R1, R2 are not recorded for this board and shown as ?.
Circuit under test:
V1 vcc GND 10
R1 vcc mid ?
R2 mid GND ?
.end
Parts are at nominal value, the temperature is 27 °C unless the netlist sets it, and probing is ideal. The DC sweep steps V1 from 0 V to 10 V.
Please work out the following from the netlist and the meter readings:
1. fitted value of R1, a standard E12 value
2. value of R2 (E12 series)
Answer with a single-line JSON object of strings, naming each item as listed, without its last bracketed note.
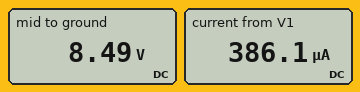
{"fitted value of R1, a standard E12 value": "3.9 kΩ", "value of R2": "22 kΩ"}
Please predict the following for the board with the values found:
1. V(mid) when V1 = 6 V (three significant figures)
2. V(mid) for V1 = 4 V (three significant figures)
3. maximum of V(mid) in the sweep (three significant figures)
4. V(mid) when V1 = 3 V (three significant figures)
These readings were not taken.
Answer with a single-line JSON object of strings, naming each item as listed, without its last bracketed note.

{"V(mid) when V1 = 6 V": "5.10 V", "V(mid) for V1 = 4 V": "3.40 V", "maximum of V(mid) in the sweep": "8.49 V", "V(mid) when V1 = 3 V": "2.55 V"}
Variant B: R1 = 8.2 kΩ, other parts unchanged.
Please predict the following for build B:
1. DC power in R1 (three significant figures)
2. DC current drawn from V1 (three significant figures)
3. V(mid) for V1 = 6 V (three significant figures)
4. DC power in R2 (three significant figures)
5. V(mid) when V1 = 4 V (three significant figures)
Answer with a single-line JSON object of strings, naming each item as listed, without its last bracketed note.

{"DC power in R1": "899 µW", "DC current drawn from V1": "331 µA", "V(mid) for V1 = 6 V": "4.37 V", "DC power in R2": "2.41 mW", "V(mid) when V1 = 4 V": "2.91 V"}
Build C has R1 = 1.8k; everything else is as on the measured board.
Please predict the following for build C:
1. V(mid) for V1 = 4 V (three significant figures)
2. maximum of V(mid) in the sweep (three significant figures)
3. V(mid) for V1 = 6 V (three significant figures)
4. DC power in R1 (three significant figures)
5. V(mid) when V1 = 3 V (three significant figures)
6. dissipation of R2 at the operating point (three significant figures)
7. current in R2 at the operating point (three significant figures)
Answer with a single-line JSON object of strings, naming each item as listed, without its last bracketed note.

{"V(mid) for V1 = 4 V": "3.70 V", "maximum of V(mid) in the sweep": "9.24 V", "V(mid) for V1 = 6 V": "5.55 V", "DC power in R1": "318 µW", "V(mid) when V1 = 3 V": "2.77 V", "dissipation of R2 at the operating point": "3.88 mW", "current in R2 at the operating point": "420 µA"}
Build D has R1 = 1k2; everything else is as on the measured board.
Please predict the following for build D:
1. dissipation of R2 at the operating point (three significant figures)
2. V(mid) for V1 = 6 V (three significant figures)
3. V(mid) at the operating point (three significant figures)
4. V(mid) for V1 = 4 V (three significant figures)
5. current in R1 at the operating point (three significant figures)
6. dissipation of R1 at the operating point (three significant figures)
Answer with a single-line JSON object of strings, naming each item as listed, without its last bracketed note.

{"dissipation of R2 at the operating point": "4.09 mW", "V(mid) for V1 = 6 V": "5.69 V", "V(mid) at the operating point": "9.48 V", "V(mid) for V1 = 4 V": "3.79 V", "current in R1 at the operating point": "431 µA", "dissipation of R1 at the operating point": "223 µW"}
